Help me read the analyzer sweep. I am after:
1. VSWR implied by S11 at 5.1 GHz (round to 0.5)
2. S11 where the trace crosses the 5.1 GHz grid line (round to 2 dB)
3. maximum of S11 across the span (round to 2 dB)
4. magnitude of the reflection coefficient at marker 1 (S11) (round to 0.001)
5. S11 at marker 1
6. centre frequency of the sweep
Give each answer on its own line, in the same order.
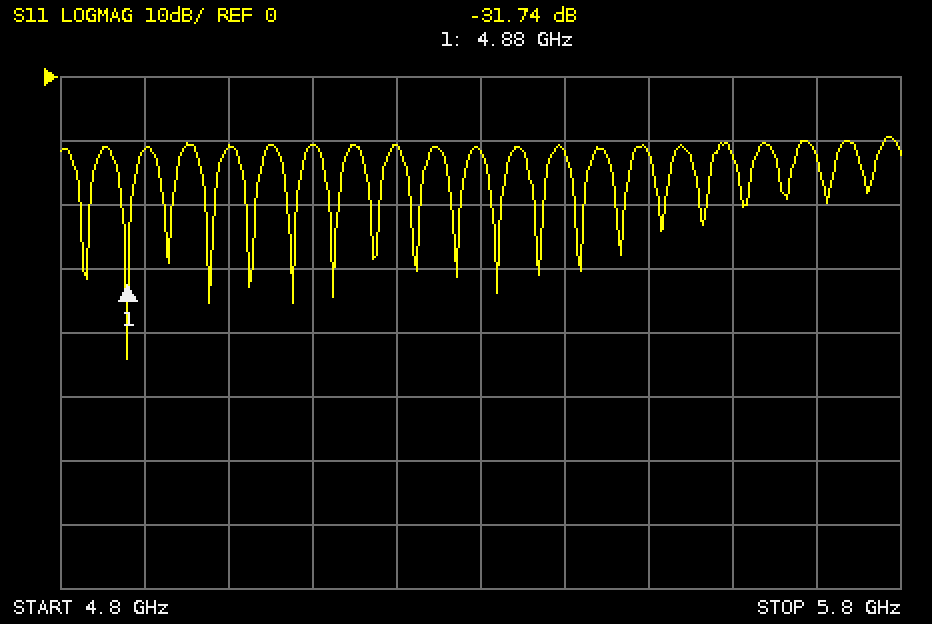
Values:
2.0
-10 dB
-10 dB
0.026
-31.74 dB
5.3 GHz
